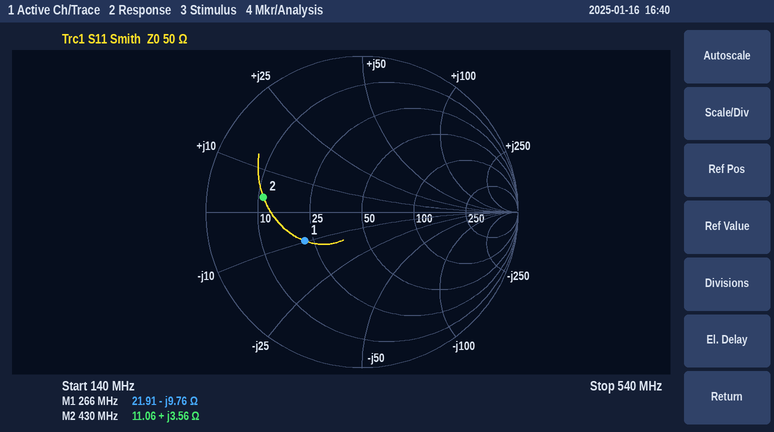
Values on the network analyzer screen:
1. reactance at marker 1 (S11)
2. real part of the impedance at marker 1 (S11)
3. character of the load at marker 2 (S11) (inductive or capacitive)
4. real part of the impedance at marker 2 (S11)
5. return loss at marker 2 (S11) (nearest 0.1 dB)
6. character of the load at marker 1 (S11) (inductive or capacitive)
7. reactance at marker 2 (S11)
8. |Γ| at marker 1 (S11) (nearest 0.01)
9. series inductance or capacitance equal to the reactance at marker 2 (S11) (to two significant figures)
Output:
-9.76 Ω
21.91 Ω
inductive
11.06 Ω
3.9 dB
capacitive
+3.56 Ω
0.41
1.3 nH
